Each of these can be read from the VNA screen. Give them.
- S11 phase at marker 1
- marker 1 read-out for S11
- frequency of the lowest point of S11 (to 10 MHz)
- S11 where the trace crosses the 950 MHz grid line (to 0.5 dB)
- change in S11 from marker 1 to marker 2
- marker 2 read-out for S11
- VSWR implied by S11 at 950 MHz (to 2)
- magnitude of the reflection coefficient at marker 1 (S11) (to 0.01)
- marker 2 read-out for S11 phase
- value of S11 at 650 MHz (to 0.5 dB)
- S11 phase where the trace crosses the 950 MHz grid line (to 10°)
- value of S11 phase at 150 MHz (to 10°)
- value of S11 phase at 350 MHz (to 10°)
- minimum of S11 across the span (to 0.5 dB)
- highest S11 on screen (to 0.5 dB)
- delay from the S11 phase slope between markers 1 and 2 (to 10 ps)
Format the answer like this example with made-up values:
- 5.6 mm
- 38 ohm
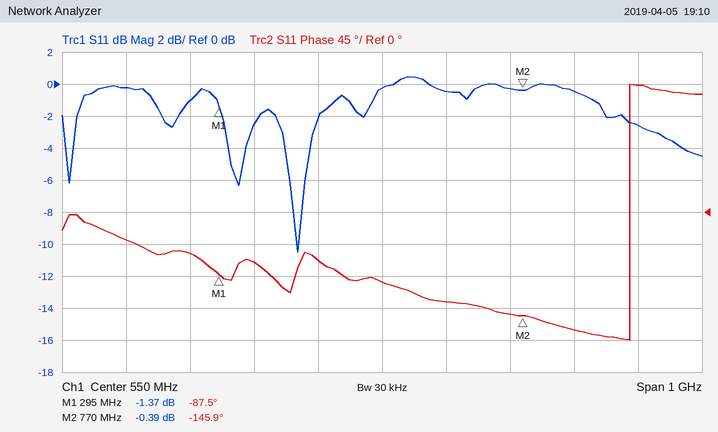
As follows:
- -87.5°
- -1.37 dB
- 420 MHz
- -2.5 dB
- 0.98 dB
- -0.39 dB
- 6
- 0.85
- -145.9°
- -0.5 dB
- 180°
- -40°
- -70°
- -10.5 dB
- 0.5 dB
- 340 ps
